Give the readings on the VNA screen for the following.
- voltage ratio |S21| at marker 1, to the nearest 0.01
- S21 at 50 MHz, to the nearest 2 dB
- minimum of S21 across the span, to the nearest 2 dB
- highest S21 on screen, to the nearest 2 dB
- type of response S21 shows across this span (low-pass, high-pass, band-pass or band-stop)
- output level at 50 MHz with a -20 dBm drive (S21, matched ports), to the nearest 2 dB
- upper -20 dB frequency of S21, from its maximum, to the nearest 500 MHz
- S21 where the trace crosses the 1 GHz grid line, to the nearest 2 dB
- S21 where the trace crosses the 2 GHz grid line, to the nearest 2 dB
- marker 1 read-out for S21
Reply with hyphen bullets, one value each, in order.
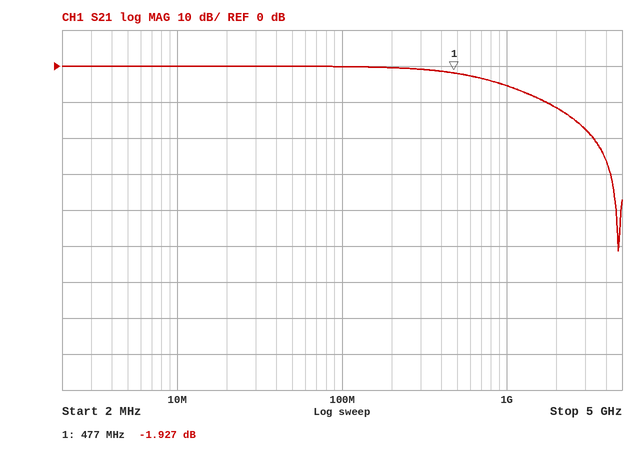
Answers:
- 0.80
- 0 dB
- -52 dB
- 0 dB
- low-pass
- -20 dBm
- 3.5 GHz
- -6 dB
- -12 dB
- -1.927 dB
